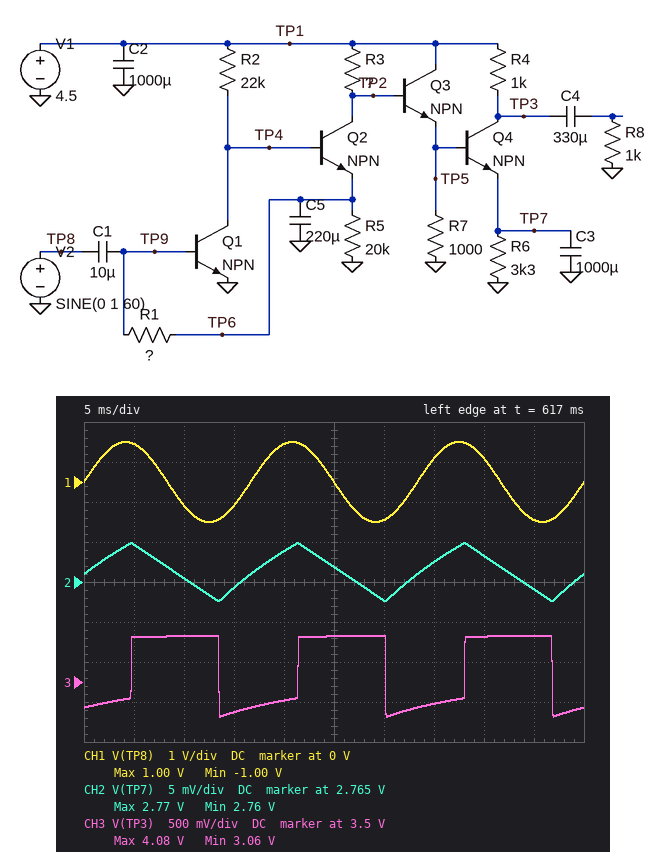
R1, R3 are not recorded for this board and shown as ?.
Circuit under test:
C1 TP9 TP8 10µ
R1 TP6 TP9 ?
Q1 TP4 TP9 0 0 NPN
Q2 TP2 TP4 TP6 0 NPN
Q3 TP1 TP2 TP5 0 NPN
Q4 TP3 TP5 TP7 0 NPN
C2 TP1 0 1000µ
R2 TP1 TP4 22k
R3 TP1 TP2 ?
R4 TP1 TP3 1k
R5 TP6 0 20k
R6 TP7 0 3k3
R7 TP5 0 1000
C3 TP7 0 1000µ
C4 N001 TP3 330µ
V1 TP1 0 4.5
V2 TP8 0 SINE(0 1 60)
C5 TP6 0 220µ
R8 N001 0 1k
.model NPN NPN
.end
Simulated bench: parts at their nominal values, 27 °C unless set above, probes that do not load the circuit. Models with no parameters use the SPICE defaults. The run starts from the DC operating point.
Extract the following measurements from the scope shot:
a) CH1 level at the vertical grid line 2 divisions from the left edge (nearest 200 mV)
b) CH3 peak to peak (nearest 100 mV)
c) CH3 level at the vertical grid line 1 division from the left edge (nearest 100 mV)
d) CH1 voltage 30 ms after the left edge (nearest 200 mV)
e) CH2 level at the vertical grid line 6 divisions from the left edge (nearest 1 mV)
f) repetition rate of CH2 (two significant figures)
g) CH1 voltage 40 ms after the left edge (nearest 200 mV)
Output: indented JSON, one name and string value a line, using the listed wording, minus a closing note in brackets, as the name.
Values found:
{
  "CH1 level at the vertical grid line 2 divisions from the left edge": "-600 mV",
  "CH3 peak to peak": "1.0 V",
  "CH3 level at the vertical grid line 1 division from the left edge": "4.1 V",
  "CH1 voltage 30 ms after the left edge": "-1.0 V",
  "CH2 level at the vertical grid line 6 divisions from the left edge": "2.763 V",
  "repetition rate of CH2": "60 Hz",
  "CH1 voltage 40 ms after the left edge": "600 mV"
}
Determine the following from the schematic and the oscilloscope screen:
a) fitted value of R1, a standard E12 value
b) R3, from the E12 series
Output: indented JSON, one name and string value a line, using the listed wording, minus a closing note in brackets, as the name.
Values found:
{
  "fitted value of R1, a standard E12 value": "56 Ω",
  "R3, from the E12 series": "3.9 kΩ"
}
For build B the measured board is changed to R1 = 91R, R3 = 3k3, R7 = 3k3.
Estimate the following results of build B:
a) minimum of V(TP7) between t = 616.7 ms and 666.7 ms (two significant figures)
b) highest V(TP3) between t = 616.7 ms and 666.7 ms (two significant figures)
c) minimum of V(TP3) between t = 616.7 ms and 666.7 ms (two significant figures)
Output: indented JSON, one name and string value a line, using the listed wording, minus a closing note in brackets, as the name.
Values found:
{
  "minimum of V(TP7) between t = 616.7 ms and 666.7 ms": "2.9 V",
  "highest V(TP3) between t = 616.7 ms and 666.7 ms": "4.1 V",
  "minimum of V(TP3) between t = 616.7 ms and 666.7 ms": "3.0 V"
}
